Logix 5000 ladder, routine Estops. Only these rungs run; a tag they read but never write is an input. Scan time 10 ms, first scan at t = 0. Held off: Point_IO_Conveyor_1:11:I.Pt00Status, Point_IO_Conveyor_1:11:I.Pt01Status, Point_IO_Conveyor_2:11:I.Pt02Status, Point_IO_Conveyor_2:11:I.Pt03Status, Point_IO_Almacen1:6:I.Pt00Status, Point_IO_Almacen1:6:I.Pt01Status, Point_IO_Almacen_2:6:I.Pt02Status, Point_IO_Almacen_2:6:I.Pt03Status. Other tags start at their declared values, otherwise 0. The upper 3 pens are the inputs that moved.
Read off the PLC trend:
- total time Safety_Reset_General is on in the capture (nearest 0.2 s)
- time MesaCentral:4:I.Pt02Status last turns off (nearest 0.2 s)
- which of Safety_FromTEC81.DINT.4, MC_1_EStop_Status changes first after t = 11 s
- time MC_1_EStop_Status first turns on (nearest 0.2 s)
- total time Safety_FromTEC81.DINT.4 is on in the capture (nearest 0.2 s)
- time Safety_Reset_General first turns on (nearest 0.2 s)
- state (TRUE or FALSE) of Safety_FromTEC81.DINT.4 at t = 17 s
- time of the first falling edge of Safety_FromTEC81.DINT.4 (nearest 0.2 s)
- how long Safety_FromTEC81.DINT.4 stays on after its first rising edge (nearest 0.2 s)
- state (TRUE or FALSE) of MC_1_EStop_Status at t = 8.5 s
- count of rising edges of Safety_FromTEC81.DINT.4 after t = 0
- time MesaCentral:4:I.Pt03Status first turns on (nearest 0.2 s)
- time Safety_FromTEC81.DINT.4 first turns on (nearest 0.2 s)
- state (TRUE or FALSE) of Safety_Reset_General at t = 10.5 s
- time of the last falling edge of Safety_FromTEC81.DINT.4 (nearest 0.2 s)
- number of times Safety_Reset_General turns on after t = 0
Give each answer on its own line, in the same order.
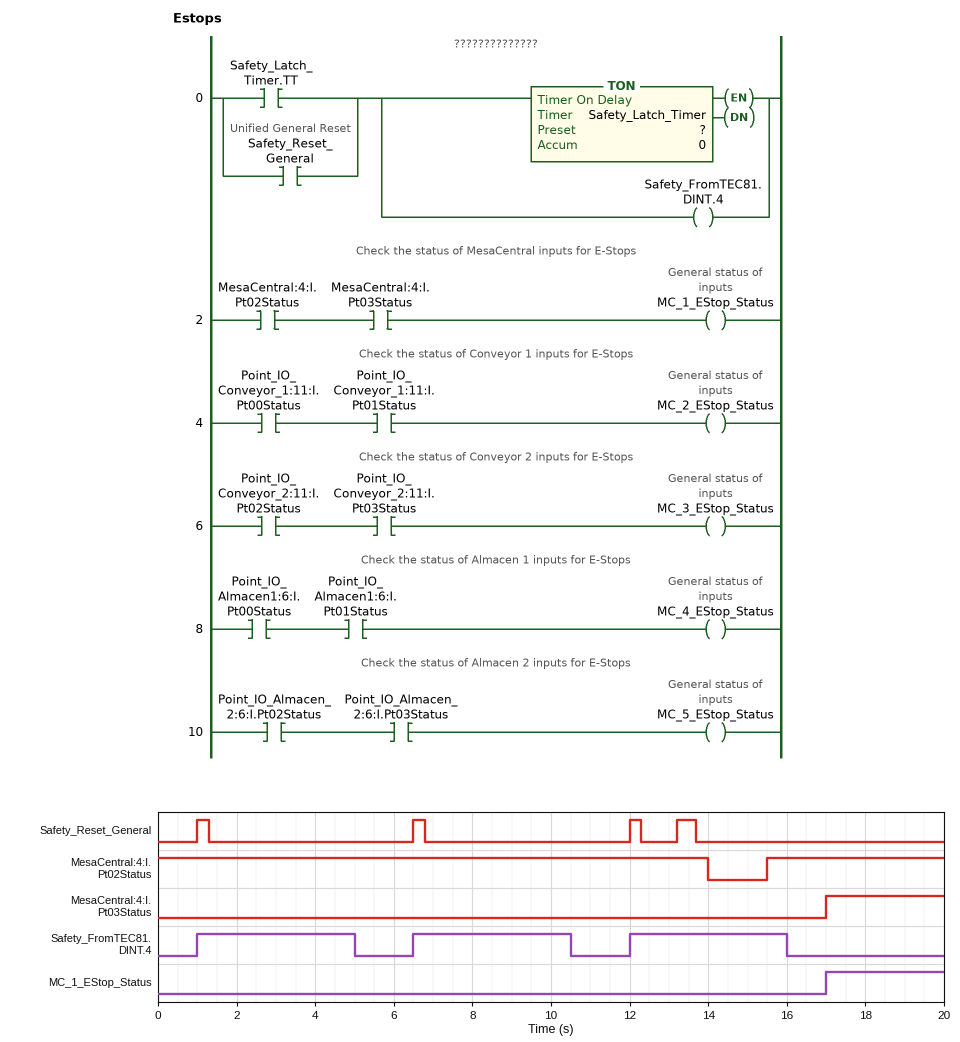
1.4 s
14.0 s
Safety_FromTEC81.DINT.4
17.0 s
12.0 s
1.0 s
FALSE
5.0 s
4.0 s
FALSE
3
17.0 s
1.0 s
FALSE
16.0 s
4
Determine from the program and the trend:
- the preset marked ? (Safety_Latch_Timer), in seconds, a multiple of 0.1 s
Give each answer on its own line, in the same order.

4.0 s
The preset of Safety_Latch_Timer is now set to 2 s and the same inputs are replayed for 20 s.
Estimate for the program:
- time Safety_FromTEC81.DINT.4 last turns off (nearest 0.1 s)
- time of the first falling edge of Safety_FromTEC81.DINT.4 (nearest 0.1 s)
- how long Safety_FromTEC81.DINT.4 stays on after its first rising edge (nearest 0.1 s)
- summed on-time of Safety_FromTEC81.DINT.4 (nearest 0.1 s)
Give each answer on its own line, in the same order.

14.0 s
3.0 s
2.0 s
6.0 s
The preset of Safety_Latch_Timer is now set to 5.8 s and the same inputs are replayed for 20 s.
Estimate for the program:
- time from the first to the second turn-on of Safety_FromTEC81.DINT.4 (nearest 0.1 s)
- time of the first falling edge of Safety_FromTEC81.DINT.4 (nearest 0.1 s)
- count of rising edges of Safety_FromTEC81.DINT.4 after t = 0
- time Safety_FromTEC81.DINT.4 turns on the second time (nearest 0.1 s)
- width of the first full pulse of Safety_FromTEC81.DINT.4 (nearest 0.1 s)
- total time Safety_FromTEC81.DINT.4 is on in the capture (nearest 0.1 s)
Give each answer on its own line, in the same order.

11.0 s
6.8 s
2
12.0 s
5.8 s
11.6 s
